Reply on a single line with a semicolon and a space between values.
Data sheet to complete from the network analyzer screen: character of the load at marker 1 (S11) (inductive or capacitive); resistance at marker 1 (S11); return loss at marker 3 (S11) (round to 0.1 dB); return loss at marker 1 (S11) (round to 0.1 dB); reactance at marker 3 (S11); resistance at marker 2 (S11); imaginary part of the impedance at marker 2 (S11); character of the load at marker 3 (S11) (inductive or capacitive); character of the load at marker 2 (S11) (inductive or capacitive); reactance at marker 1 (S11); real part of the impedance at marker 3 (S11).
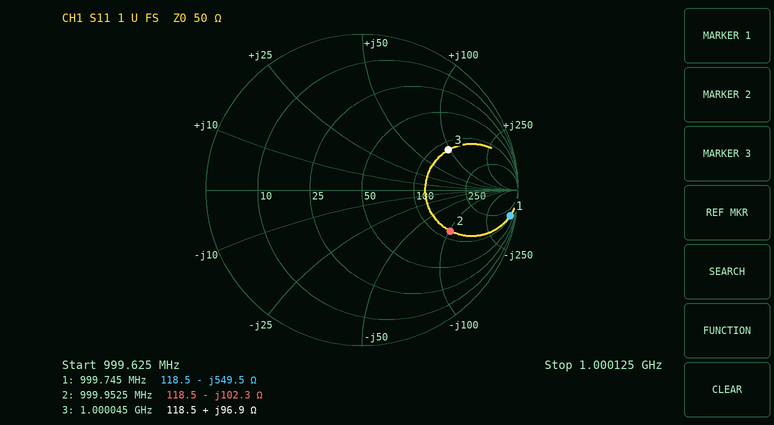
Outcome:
capacitive; 118.5 Ω; 4.3 dB; 0.3 dB; +96.9 Ω; 118.5 Ω; -102.3 Ω; inductive; capacitive; -549.5 Ω; 118.5 Ω
